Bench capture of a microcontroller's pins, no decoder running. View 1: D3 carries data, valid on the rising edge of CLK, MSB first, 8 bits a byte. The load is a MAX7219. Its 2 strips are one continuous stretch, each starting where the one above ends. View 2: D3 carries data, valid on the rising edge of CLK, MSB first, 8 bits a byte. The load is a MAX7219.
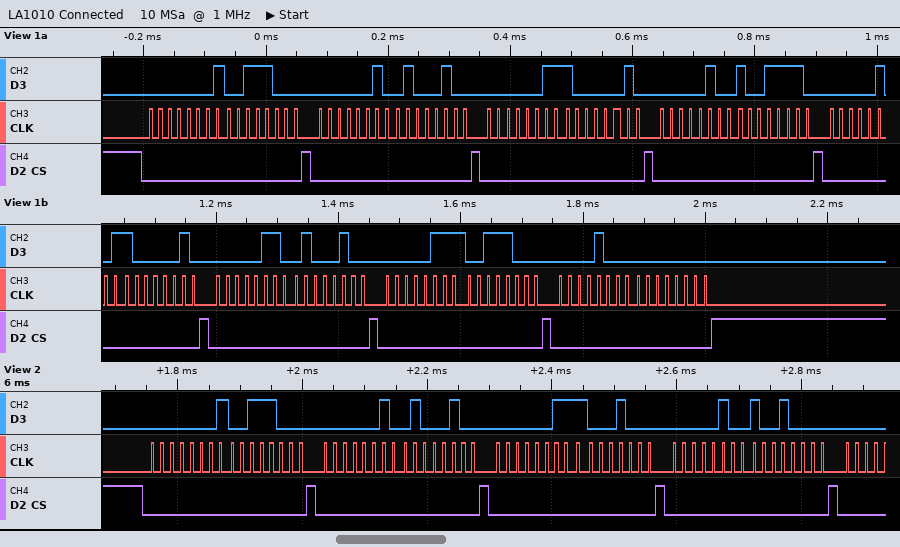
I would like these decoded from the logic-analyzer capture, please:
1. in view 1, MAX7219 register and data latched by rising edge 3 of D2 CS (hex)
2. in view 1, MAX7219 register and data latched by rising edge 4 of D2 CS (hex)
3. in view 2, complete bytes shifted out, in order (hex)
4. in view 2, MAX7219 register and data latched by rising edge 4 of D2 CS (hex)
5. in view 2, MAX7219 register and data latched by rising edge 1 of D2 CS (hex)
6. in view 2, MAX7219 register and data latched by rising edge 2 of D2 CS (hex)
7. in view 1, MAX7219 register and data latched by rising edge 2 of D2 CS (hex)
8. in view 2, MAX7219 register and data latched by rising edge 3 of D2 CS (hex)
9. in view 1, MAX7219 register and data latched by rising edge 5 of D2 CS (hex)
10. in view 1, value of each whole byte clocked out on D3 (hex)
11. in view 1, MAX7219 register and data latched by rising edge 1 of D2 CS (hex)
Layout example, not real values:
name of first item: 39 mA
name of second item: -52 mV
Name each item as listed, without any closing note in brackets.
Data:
in view 1, MAX7219 register and data latched by rising edge 3 of D2 CS: register 0x3, data 0x82
in view 1, MAX7219 register and data latched by rising edge 4 of D2 CS: register 0x4, data 0x9E
in view 2, complete bytes shifted out, in order: 01 38 02 44 03 88 04 90
in view 2, MAX7219 register and data latched by rising edge 4 of D2 CS: register 0x4, data 0x90
in view 2, MAX7219 register and data latched by rising edge 1 of D2 CS: register 0x1, data 0x38
in view 2, MAX7219 register and data latched by rising edge 2 of D2 CS: register 0x2, data 0x44
in view 1, MAX7219 register and data latched by rising edge 2 of D2 CS: register 0x2, data 0x44
in view 2, MAX7219 register and data latched by rising edge 3 of D2 CS: register 0x3, data 0x88
in view 1, MAX7219 register and data latched by rising edge 5 of D2 CS: register 0x5, data 0x82
in view 1, value of each whole byte clocked out on D3: 0x01 0x38 0x02 0x44 0x03 0x82 0x04 0x9E 0x05 0x82 0x06 0x44 0x07 0x38 0x08 0x00
in view 1, MAX7219 register and data latched by rising edge 1 of D2 CS: register 0x1, data 0x38
